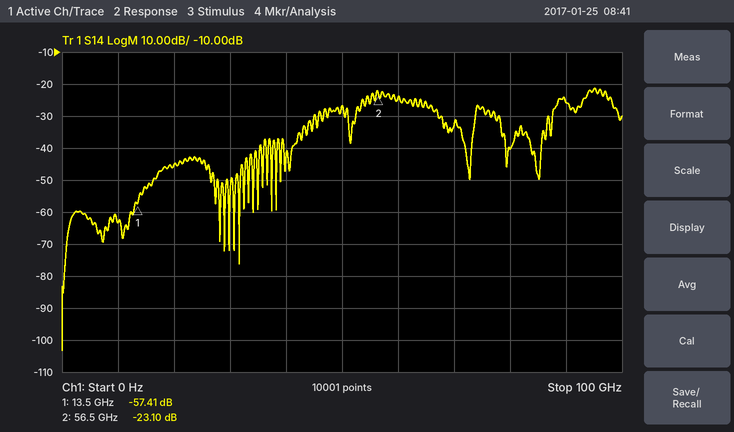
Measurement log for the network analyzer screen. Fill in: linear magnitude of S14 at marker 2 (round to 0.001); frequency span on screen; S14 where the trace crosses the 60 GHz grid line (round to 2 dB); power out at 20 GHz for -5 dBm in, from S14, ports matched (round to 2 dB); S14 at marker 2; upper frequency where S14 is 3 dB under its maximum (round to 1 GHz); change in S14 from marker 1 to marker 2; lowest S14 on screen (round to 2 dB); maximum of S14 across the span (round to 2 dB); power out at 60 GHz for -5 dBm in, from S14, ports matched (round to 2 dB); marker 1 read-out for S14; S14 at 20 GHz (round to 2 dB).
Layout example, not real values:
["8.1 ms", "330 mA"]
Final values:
["0.070", "100 GHz", "-24 dB", "-50 dBm", "-23.10 dB", "97 GHz", "34.31 dB", "-104 dB", "-22 dB", "-30 dBm", "-57.41 dB", "-46 dB"]
